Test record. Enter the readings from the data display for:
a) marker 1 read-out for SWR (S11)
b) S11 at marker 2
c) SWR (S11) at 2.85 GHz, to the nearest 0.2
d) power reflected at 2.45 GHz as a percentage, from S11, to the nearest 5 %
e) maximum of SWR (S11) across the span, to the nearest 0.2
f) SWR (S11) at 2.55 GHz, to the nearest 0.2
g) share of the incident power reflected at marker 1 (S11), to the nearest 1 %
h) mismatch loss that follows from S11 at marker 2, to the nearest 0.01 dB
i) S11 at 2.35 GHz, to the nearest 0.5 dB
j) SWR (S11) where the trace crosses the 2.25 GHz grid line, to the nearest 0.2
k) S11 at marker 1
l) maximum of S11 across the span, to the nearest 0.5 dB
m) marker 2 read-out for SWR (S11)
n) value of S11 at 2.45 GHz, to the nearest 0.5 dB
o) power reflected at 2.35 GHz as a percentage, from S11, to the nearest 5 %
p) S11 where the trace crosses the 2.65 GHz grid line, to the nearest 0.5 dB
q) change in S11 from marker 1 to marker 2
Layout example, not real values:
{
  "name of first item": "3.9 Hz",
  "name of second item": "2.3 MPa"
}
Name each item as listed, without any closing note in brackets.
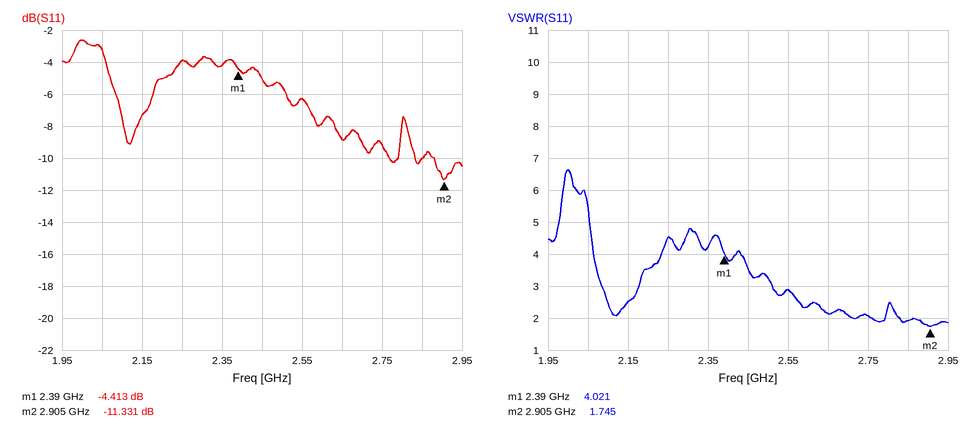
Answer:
{
  "marker 1 read-out for SWR": "4.021",
  "S11 at marker 2": "-11.331 dB",
  "SWR (S11) at 2.85 GHz, to the nearest 0.2": "2.0",
  "power reflected at 2.45 GHz as a percentage, from S11, to the nearest 5 %": "30 %",
  "maximum of SWR (S11) across the span, to the nearest 0.2": "6.6",
  "SWR (S11) at 2.55 GHz, to the nearest 0.2": "2.8",
  "share of the incident power reflected at marker 1 (S11), to the nearest 1 %": "36 %",
  "mismatch loss that follows from S11 at marker 2, to the nearest 0.01 dB": "0.33 dB",
  "S11 at 2.35 GHz, to the nearest 0.5 dB": "-4.0 dB",
  "SWR (S11) where the trace crosses the 2.25 GHz grid line, to the nearest 0.2": "4.6",
  "S11 at marker 1": "-4.413 dB",
  "maximum of S11 across the span, to the nearest 0.5 dB": "-2.5 dB",
  "marker 2 read-out for SWR": "1.745",
  "value of S11 at 2.45 GHz, to the nearest 0.5 dB": "-5.0 dB",
  "power reflected at 2.35 GHz as a percentage, from S11, to the nearest 5 %": "40 %",
  "S11 where the trace crosses the 2.65 GHz grid line, to the nearest 0.5 dB": "-9.0 dB",
  "change in S11 from marker 1 to marker 2": "-6.918 dB"
}
